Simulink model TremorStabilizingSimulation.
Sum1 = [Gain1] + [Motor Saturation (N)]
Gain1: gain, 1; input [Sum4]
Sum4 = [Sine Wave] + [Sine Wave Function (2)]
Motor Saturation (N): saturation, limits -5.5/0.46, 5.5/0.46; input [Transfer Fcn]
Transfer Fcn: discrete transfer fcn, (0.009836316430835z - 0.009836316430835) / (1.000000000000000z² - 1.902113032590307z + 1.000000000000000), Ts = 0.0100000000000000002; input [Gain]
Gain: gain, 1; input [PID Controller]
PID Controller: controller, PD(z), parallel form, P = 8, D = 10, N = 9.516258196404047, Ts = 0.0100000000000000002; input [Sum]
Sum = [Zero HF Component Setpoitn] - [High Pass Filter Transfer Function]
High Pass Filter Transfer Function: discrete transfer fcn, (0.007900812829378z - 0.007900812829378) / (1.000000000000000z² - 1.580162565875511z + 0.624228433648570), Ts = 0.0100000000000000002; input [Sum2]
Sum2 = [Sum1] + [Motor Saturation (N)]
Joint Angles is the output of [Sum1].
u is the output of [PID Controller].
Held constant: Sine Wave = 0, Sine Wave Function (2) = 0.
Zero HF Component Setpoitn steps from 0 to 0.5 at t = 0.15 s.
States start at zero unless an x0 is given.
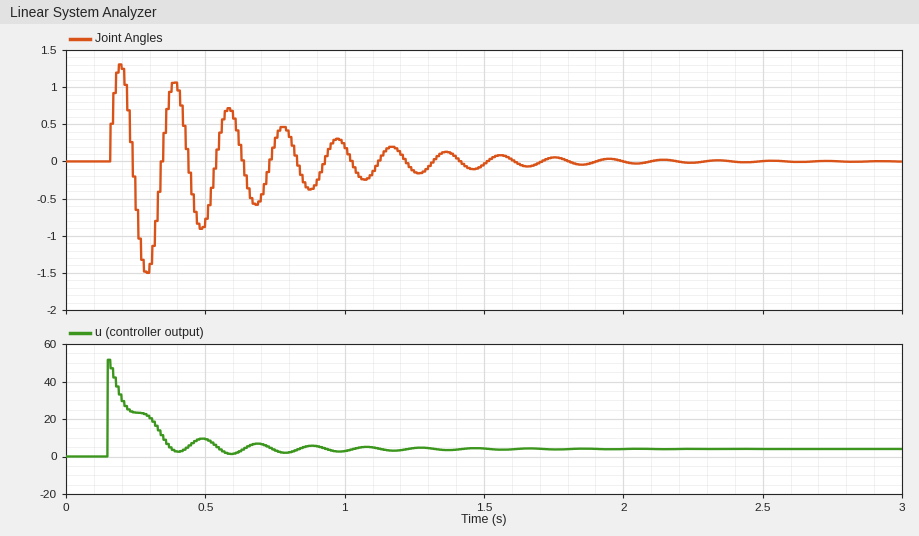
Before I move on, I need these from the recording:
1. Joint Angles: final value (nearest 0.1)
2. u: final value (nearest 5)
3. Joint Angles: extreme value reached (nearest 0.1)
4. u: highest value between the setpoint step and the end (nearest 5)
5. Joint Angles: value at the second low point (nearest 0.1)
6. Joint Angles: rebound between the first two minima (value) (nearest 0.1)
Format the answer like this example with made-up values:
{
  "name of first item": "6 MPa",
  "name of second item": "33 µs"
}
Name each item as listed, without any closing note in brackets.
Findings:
{
  "Joint Angles: final value": "0.0",
  "u: final value": "5",
  "Joint Angles: extreme value reached": "-1.5",
  "u: highest value between the setpoint step and the end": "50",
  "Joint Angles: value at the second low point": "-0.9",
  "Joint Angles: rebound between the first two minima (value)": "1.1"
}
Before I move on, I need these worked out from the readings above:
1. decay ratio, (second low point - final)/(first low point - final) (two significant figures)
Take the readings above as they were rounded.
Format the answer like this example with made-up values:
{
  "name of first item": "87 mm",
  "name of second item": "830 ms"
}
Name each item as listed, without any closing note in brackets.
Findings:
{
  "decay ratio, (second low point - final)/(first low point - final)": "0.60"
}
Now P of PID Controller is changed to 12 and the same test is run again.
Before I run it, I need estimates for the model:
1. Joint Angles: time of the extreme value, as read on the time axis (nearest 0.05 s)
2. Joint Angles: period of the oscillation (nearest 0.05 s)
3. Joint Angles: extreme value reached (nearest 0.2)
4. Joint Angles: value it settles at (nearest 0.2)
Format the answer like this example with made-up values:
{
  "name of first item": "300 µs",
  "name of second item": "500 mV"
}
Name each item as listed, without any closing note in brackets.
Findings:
{
  "Joint Angles: time of the extreme value, as read on the time axis": "0.30 s",
  "Joint Angles: period of the oscillation": "0.20 s",
  "Joint Angles: extreme value reached": "-1.6",
  "Joint Angles: value it settles at": "0.0"
}
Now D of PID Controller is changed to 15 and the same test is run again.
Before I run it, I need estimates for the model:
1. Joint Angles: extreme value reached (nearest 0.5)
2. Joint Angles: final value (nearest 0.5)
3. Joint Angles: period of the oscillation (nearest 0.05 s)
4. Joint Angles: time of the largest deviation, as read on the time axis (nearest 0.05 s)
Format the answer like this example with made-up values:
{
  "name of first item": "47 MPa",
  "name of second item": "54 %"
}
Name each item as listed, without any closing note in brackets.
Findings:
{
  "Joint Angles: extreme value reached": "-2.0",
  "Joint Angles: final value": "0.0",
  "Joint Angles: period of the oscillation": "0.20 s",
  "Joint Angles: time of the largest deviation, as read on the time axis": "0.30 s"
}
